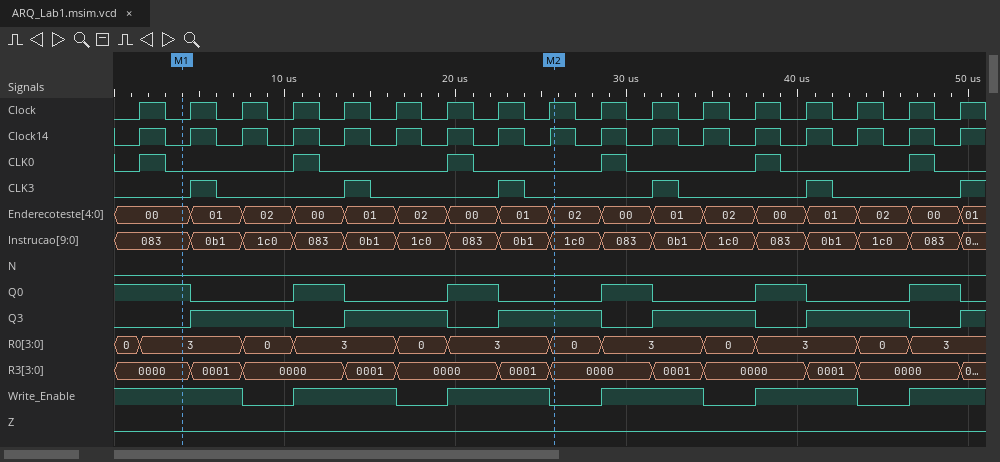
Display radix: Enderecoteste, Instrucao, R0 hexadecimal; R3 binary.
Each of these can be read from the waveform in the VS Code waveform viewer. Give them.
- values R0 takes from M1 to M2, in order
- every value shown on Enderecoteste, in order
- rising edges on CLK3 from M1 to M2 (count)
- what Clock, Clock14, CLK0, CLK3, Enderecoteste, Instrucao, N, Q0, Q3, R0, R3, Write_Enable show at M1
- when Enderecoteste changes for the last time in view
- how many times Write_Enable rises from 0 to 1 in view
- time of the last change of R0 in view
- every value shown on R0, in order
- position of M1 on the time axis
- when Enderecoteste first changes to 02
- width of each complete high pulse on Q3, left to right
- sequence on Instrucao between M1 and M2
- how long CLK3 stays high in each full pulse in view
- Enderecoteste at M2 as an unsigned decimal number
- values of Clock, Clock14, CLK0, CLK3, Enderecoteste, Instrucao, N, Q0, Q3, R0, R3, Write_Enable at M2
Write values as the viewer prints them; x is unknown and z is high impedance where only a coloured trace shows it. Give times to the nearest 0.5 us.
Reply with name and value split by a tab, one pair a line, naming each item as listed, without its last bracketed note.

values R0 takes from M1 to M2, in order	3, 0, 3, 0, 3, 0
every value shown on Enderecoteste, in order	00, 01, 02, 00, 01, 02, 00, 01, 02, 00, 01, 02, 00, 01, 02, 00, 01
rising edges on CLK3 from M1 to M2	3
what Clock, Clock14, CLK0, CLK3, Enderecoteste, Instrucao, N, Q0, Q3, R0, R3, Write_Enable show at M1	Clock=0, Clock14=0, CLK0=0, CLK3=0, Enderecoteste=00, Instrucao=083, N=0, Q0=1, Q3=0, R0=3, R3=0000, Write_Enable=1
when Enderecoteste changes for the last time in view	49.5 us
how many times Write_Enable rises from 0 to 1 in view	5
time of the last change of R0 in view	46.5 us
every value shown on R0, in order	0, 3, 0, 3, 0, 3, 0, 3, 0, 3, 0, 3
position of M1 on the time axis	4 us
when Enderecoteste first changes to 02	7.5 us
width of each complete high pulse on Q3, left to right	6 us, 6 us, 6 us, 6 us, 6 us
sequence on Instrucao between M1 and M2	083, 0b1, 1c0, 083, 0b1, 1c0, 083, 0b1, 1c0
how long CLK3 stays high in each full pulse in view	1.5 us, 1.5 us, 1.5 us, 1.5 us, 1.5 us
Enderecoteste at M2 as an unsigned decimal number	2
values of Clock, Clock14, CLK0, CLK3, Enderecoteste, Instrucao, N, Q0, Q3, R0, R3, Write_Enable at M2	Clock=1, Clock14=1, CLK0=0, CLK3=0, Enderecoteste=02, Instrucao=1c0, N=0, Q0=0, Q3=1, R0=0, R3=0000, Write_Enable=0
